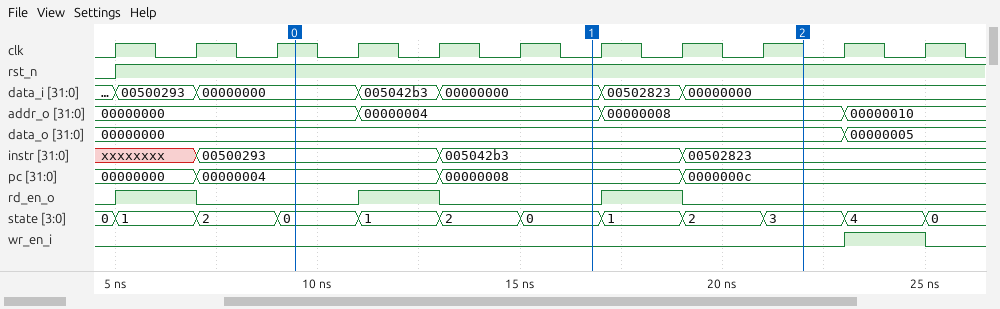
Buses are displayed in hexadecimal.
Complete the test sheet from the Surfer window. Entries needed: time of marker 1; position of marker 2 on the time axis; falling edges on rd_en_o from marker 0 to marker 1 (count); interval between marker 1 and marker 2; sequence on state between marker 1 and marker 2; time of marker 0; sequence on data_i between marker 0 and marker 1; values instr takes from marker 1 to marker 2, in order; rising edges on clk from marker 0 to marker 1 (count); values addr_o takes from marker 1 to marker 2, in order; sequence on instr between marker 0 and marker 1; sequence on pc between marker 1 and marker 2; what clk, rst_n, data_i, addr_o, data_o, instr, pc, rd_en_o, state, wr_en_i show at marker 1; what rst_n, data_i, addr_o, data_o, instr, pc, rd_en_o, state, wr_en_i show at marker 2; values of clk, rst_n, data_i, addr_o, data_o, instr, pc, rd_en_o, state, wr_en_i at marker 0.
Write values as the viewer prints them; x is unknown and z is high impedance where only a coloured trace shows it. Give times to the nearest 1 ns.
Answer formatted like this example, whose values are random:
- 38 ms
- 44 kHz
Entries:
- 17 ns
- 22 ns
- 1
- 5 ns
- 0, 1, 2, 3
- 9 ns
- 00000000, 005042b3, 00000000
- 005042b3, 00502823
- 3
- 00000004, 00000008
- 00500293, 005042b3
- 00000008, 0000000c
- clk=0, rst_n=1, data_i=00000000, addr_o=00000004, data_o=00000000, instr=005042b3, pc=00000008, rd_en_o=0, state=0, wr_en_i=0
- rst_n=1, data_i=00000000, addr_o=00000008, data_o=00000000, instr=00502823, pc=0000000c, rd_en_o=0, state=3, wr_en_i=0
- clk=1, rst_n=1, data_i=00000000, addr_o=00000000, data_o=00000000, instr=00500293, pc=00000004, rd_en_o=0, state=0, wr_en_i=0
